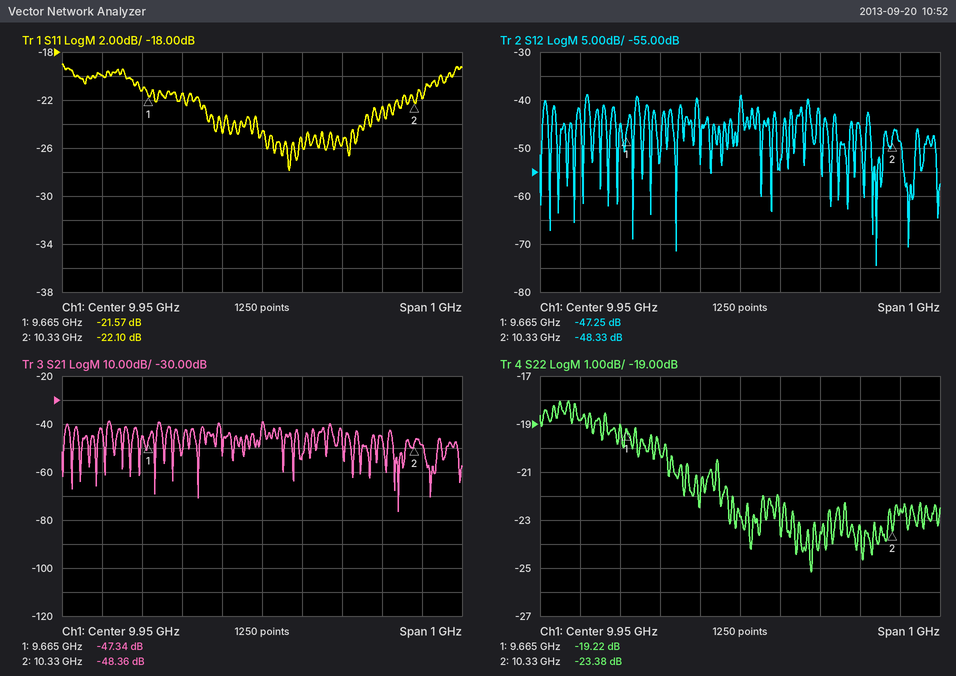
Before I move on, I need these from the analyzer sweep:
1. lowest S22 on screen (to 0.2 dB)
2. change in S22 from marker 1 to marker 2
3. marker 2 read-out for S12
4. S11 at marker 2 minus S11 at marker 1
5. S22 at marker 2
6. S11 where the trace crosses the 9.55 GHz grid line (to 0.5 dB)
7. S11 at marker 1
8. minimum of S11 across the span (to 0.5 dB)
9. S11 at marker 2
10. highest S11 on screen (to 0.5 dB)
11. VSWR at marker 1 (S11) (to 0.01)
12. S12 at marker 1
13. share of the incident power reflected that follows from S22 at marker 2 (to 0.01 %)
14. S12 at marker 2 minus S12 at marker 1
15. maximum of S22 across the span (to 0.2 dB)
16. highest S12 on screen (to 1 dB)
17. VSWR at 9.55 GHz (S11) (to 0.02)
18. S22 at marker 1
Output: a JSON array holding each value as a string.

["-25.2 dB", "-4.16 dB", "-48.33 dB", "-0.53 dB", "-23.38 dB", "-20.0 dB", "-21.57 dB", "-28.0 dB", "-22.10 dB", "-19.0 dB", "1.18", "-47.25 dB", "0.46 %", "-1.08 dB", "-18.0 dB", "-39 dB", "1.22", "-19.22 dB"]
